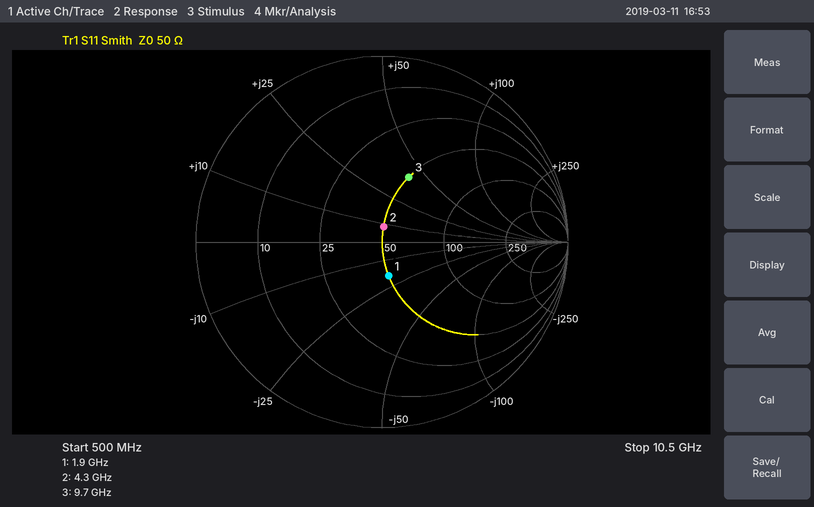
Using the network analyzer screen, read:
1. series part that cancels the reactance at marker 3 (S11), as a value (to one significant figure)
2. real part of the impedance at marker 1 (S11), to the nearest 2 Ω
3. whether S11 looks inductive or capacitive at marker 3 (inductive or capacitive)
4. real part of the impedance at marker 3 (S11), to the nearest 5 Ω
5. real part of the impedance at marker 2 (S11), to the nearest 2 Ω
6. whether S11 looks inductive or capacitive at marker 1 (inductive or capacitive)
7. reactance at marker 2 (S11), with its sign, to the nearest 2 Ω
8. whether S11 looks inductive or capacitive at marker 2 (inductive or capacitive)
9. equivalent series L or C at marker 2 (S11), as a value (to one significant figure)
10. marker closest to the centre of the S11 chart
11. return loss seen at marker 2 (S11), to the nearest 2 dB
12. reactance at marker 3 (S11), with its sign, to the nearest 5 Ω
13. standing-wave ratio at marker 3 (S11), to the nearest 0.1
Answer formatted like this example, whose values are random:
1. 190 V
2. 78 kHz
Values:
1. 400 fF
2. 50 Ω
3. inductive
4. 50 Ω
5. 50 Ω
6. capacitive
7. +8 Ω
8. inductive
9. 300 pH
10. marker 2
11. 22 dB
12. +40 Ω
13. 2.2
